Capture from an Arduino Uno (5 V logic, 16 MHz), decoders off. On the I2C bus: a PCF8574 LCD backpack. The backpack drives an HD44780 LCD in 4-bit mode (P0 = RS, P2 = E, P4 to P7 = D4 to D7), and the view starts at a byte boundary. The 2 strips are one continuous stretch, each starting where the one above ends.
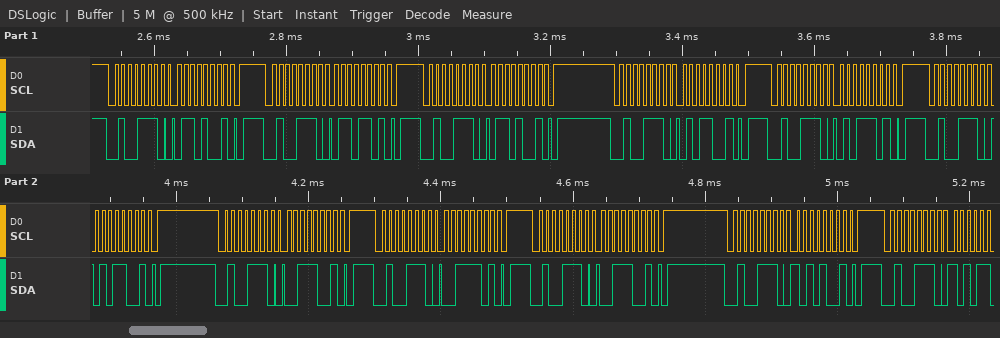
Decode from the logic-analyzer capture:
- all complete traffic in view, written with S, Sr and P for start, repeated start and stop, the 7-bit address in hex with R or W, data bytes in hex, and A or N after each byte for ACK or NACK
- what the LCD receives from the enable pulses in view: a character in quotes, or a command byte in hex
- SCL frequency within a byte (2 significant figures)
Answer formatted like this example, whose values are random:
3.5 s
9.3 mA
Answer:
S 27W A 69 A P S 27W A 6D A P S 27W A 69 A P S 27W A 59 A P S 27W A 5D A P S 27W A 59 A P S 27W A 39 A P S 27W A 3D A P S 27W A 39 A P S 27W A A9 A P S 27W A
'e'
100 kHz
